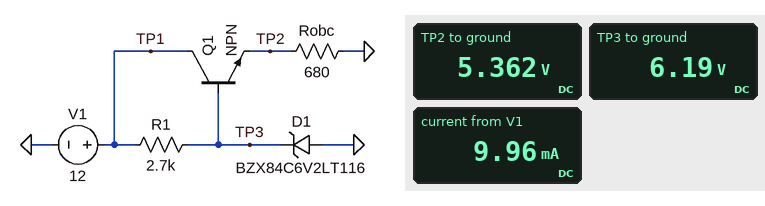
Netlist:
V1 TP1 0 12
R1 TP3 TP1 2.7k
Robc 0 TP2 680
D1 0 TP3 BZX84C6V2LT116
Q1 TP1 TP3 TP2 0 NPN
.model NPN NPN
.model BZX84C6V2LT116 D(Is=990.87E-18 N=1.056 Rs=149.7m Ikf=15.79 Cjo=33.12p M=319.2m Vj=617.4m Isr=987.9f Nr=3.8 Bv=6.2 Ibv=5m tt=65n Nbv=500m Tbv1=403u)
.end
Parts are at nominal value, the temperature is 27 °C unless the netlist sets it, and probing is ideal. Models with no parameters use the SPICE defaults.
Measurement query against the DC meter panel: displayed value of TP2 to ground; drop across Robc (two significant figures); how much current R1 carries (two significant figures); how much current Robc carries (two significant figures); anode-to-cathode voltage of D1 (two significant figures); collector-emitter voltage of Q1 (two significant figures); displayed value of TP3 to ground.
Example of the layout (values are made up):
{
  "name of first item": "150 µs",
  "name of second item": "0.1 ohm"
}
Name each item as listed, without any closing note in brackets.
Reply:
{
  "displayed value of TP2 to ground": "5.362 V",
  "drop across Robc": "5.4 V",
  "how much current R1 carries": "2.2 mA",
  "how much current Robc carries": "7.9 mA",
  "anode-to-cathode voltage of D1": "-6.2 V",
  "collector-emitter voltage of Q1": "6.6 V",
  "displayed value of TP3 to ground": "6.19 V"
}
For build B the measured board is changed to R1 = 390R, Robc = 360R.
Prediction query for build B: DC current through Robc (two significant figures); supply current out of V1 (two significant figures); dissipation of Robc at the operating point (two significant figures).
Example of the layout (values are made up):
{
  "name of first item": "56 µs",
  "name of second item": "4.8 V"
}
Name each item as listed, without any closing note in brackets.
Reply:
{
  "DC current through Robc": "15 mA",
  "supply current out of V1": "30 mA",
  "dissipation of Robc at the operating point": "80 mW"
}
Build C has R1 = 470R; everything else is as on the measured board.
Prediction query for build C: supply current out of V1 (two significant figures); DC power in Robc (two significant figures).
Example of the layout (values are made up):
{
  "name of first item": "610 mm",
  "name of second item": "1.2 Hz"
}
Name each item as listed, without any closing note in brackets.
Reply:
{
  "supply current out of V1": "20 mA",
  "DC power in Robc": "43 mW"
}
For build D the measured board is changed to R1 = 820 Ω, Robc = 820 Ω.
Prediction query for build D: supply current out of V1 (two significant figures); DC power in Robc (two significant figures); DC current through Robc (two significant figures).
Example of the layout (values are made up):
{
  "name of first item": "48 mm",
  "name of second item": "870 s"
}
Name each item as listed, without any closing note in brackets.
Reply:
{
  "supply current out of V1": "14 mA",
  "DC power in Robc": "35 mW",
  "DC current through Robc": "6.6 mA"
}
